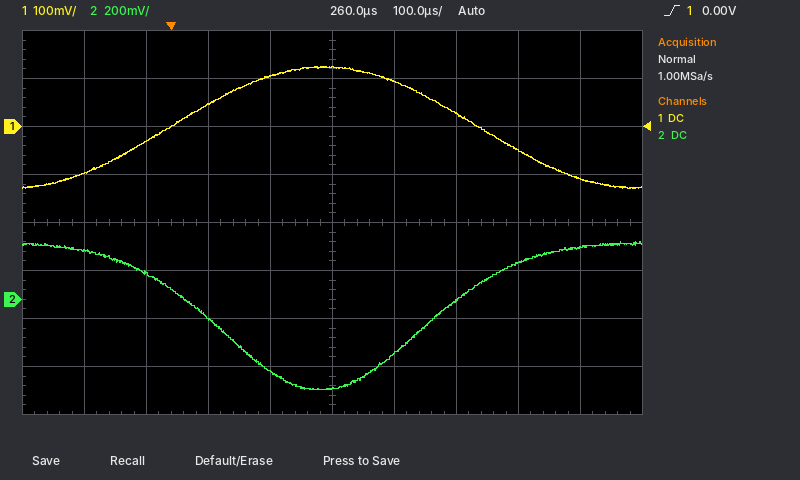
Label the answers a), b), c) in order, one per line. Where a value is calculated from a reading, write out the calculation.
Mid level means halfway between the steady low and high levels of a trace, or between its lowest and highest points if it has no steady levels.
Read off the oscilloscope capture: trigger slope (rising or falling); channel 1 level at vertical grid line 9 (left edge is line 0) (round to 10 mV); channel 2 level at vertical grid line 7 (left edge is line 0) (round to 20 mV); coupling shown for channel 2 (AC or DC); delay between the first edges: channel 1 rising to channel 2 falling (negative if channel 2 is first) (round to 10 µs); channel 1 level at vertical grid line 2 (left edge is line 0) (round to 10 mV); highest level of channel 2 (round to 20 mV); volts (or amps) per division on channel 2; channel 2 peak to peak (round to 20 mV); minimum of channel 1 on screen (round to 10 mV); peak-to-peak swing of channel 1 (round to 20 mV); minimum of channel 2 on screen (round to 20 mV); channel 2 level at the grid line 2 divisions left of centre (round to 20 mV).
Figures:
a) rising
b) -110 mV
c) 0 mV
d) DC
e) +60 µs
f) -30 mV
g) 240 mV
h) 200 mV
i) 240 mV − (-380 mV) = 620 mV
j) -130 mV
k) 260 mV
l) -380 mV
m) -80 mV
